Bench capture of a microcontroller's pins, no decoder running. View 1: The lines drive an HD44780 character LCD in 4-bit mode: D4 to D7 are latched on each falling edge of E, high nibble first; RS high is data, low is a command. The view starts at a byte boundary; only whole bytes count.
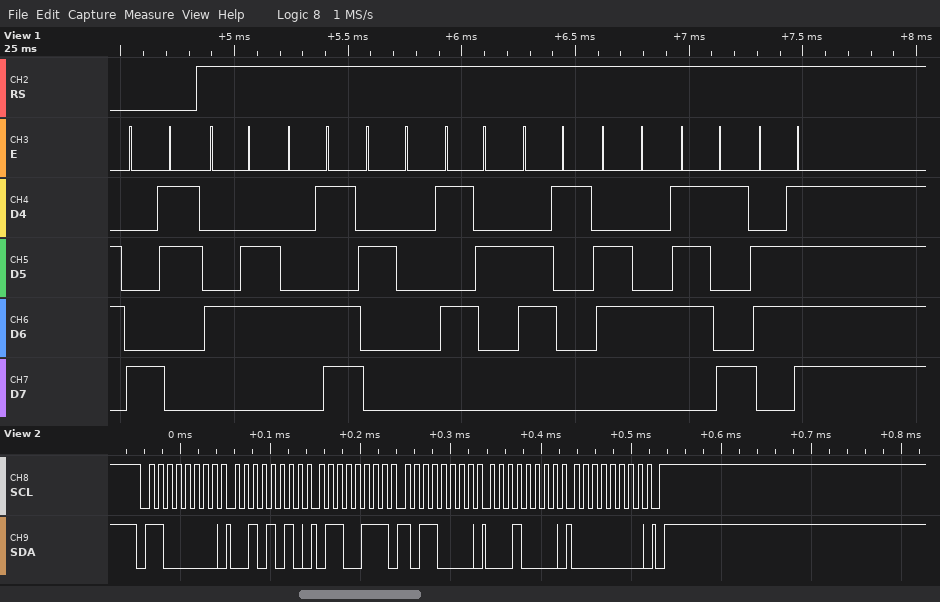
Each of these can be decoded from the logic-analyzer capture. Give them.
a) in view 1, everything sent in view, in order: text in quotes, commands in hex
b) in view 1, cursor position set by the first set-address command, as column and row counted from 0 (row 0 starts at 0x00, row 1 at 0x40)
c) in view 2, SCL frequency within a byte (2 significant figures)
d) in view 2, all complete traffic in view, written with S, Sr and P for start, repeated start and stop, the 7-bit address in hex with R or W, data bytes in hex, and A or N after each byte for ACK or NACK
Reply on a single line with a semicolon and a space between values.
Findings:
0x83 "FM Radyo"; column 3, row 0; 100 kHz; S 60W A 2A A 67 A B0 A 10 A 00 A P
